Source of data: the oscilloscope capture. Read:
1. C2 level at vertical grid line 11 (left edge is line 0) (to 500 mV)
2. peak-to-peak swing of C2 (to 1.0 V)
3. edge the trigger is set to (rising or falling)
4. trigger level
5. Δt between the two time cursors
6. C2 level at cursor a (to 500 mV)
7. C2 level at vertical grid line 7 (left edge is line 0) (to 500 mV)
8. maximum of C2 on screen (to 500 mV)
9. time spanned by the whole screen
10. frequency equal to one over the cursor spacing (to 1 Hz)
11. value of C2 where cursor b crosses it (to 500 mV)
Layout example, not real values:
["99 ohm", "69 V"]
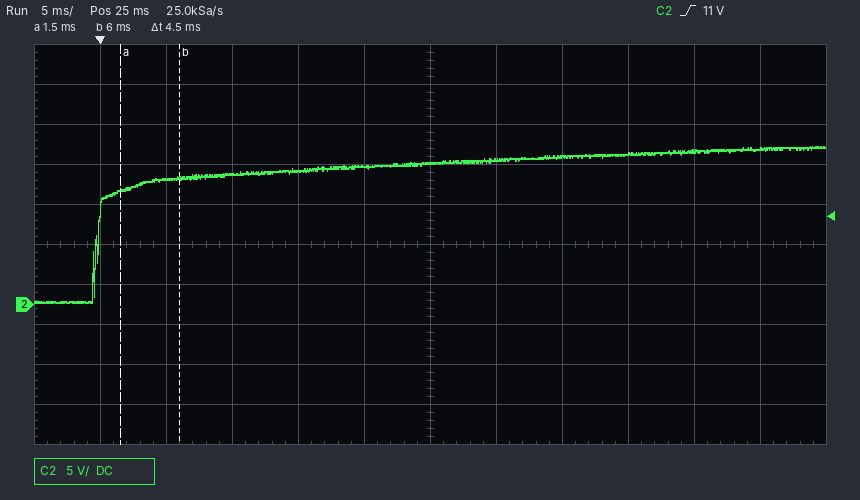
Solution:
["19.5 V", "20.0 V", "rising", "11 V", "4.5 ms", "14.0 V", "18.0 V", "20.0 V", "60 ms", "222 Hz", "16.0 V"]
